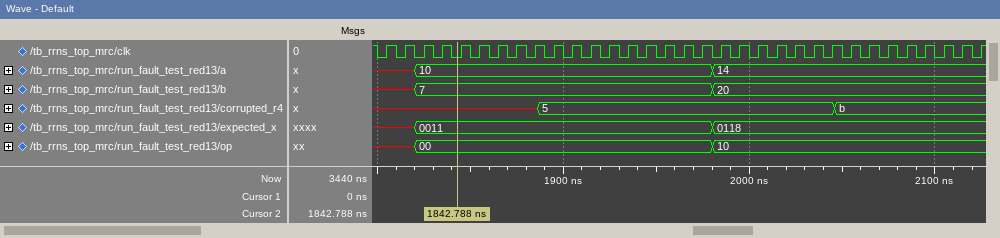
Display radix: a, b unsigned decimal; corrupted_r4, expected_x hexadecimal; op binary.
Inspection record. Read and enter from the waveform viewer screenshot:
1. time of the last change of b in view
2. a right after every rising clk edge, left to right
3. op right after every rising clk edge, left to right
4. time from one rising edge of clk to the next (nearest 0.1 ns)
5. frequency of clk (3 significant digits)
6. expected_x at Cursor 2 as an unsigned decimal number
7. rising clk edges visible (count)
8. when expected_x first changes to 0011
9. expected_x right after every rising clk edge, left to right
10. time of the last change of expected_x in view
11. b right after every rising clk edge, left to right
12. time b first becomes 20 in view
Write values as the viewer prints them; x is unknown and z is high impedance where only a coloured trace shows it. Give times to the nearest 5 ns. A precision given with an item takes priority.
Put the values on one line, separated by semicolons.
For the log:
1980 ns; x, x, 10, 10, 10, 10, 10, 10, 10, 10, 10, 10, 10, 10, 10, 10, 10, 10, 14, 14, 14, 14, 14, 14, 14, 14, 14, 14, 14, 14, 14, 14, 14; x, x, 00, 00, 00, 00, 00, 00, 00, 00, 00, 00, 00, 00, 00, 00, 00, 00, 10, 10, 10, 10, 10, 10, 10, 10, 10, 10, 10, 10, 10, 10, 10; 10 ns; 100 MHz; 17; 33; 1820 ns; x, x, 0011, 0011, 0011, 0011, 0011, 0011, 0011, 0011, 0011, 0011, 0011, 0011, 0011, 0011, 0011, 0011, 0118, 0118, 0118, 0118, 0118, 0118, 0118, 0118, 0118, 0118, 0118, 0118, 0118, 0118, 0118; 1980 ns; x, x, 7, 7, 7, 7, 7, 7, 7, 7, 7, 7, 7, 7, 7, 7, 7, 7, 20, 20, 20, 20, 20, 20, 20, 20, 20, 20, 20, 20, 20, 20, 20; 1980 ns
